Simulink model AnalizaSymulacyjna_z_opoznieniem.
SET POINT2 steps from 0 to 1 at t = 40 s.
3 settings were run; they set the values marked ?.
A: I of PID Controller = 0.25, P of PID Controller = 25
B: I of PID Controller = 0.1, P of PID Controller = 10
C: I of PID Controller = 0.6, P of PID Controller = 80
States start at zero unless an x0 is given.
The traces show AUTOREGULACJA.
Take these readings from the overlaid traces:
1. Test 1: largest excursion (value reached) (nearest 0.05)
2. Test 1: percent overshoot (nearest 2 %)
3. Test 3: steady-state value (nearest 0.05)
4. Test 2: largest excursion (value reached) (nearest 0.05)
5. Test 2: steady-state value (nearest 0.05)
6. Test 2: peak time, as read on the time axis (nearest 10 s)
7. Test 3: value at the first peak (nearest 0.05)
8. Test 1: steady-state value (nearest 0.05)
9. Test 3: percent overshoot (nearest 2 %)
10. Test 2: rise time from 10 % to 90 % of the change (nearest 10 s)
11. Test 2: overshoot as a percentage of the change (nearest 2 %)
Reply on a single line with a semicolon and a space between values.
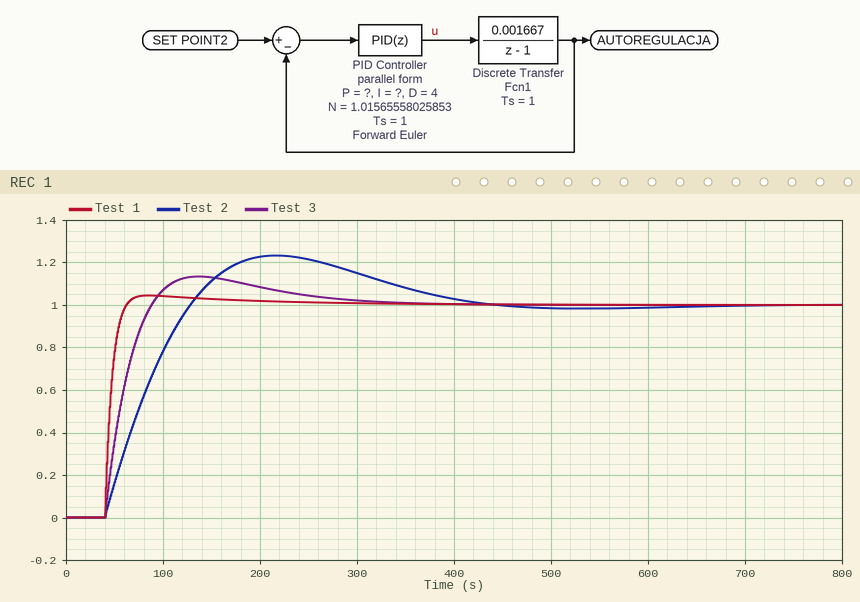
1.05; 4 %; 1.00; 1.25; 1.00; 220 s; 1.15; 1.00; 14 %; 70 s; 24 %
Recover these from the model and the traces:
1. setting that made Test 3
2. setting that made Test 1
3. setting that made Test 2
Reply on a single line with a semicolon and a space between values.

A; C; B
